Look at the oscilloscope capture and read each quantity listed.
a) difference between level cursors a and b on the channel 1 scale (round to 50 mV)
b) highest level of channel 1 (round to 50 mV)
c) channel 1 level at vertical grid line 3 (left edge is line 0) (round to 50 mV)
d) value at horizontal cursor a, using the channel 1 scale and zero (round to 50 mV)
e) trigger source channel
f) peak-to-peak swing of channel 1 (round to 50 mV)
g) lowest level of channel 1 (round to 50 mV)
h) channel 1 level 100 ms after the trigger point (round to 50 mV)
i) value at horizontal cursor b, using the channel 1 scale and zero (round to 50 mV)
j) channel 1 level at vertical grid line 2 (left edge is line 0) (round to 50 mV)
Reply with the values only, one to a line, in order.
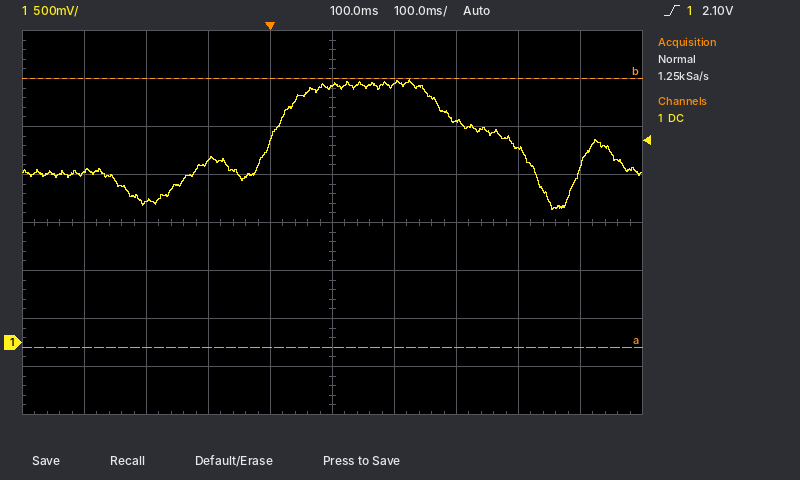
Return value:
2.80 V
2.75 V
1.90 V
-50 mV
channel 1
1.35 V
1.40 V
2.65 V
2.75 V
1.45 V
